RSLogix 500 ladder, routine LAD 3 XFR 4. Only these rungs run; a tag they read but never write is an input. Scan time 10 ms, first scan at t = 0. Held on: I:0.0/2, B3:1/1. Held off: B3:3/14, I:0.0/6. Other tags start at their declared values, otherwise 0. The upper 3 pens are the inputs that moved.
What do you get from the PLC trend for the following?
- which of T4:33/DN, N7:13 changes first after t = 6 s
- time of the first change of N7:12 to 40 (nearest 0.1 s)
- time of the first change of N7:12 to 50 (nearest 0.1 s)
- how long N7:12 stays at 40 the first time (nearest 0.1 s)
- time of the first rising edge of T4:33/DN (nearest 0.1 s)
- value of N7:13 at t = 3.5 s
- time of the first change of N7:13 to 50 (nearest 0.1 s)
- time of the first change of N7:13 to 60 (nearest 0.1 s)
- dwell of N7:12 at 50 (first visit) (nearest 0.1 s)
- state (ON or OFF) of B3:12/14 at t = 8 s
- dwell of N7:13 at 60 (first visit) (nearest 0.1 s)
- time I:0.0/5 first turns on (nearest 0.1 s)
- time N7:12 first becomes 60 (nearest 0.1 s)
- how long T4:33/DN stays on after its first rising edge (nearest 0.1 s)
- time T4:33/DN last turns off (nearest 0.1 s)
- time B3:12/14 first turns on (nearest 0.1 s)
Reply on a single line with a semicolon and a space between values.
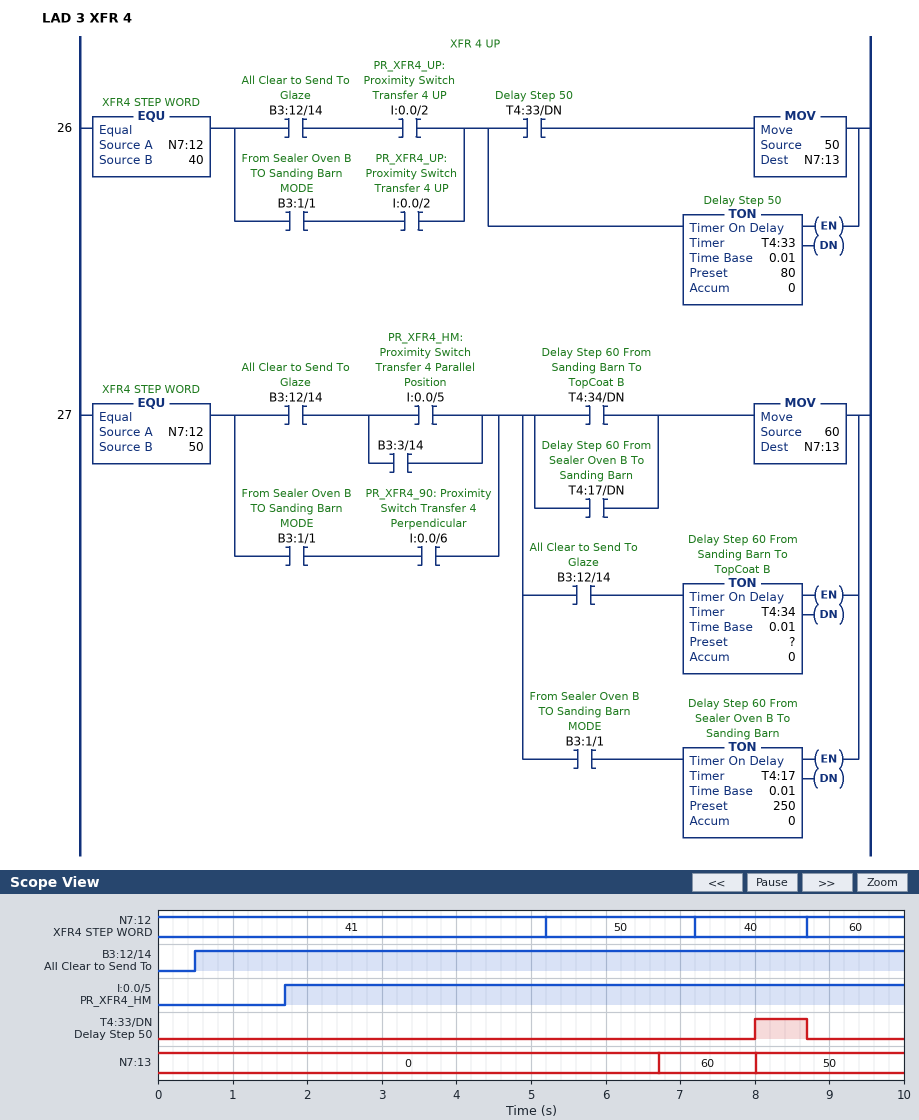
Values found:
N7:13; 7.2 s; 5.2 s; 1.5 s; 8.0 s; 0; 8.0 s; 6.7 s; 2.0 s; ON; 1.3 s; 1.7 s; 8.7 s; 0.7 s; 8.7 s; 0.5 s
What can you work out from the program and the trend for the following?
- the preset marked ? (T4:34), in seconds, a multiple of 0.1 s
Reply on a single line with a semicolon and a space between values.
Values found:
1.5 s
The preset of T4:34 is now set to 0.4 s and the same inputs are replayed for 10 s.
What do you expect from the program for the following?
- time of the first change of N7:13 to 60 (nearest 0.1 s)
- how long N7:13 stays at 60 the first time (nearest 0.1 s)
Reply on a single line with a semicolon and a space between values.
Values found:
5.6 s; 2.4 s
